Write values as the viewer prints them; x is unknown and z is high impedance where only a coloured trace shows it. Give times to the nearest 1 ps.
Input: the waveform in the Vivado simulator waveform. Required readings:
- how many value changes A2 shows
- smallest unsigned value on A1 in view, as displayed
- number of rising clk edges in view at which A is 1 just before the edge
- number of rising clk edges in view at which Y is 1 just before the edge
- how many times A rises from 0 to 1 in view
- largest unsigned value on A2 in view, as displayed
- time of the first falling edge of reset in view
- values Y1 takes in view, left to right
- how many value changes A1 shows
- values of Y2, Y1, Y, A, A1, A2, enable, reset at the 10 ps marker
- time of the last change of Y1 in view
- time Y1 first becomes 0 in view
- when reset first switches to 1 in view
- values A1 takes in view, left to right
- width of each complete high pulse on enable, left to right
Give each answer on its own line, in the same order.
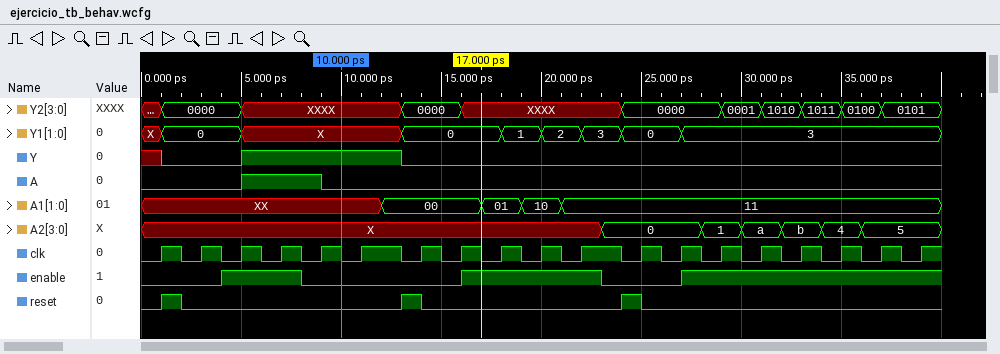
6
00
2
3
1
b
2 ps
X, 0, X, 0, 1, 2, 3, 0, 3
4
Y2=XXXX, Y1=X, Y=1, A=0, A1=XX, A2=X, enable=0, reset=0
27 ps
1 ps
1 ps
XX, 00, 01, 10, 11
4 ps, 7 ps
